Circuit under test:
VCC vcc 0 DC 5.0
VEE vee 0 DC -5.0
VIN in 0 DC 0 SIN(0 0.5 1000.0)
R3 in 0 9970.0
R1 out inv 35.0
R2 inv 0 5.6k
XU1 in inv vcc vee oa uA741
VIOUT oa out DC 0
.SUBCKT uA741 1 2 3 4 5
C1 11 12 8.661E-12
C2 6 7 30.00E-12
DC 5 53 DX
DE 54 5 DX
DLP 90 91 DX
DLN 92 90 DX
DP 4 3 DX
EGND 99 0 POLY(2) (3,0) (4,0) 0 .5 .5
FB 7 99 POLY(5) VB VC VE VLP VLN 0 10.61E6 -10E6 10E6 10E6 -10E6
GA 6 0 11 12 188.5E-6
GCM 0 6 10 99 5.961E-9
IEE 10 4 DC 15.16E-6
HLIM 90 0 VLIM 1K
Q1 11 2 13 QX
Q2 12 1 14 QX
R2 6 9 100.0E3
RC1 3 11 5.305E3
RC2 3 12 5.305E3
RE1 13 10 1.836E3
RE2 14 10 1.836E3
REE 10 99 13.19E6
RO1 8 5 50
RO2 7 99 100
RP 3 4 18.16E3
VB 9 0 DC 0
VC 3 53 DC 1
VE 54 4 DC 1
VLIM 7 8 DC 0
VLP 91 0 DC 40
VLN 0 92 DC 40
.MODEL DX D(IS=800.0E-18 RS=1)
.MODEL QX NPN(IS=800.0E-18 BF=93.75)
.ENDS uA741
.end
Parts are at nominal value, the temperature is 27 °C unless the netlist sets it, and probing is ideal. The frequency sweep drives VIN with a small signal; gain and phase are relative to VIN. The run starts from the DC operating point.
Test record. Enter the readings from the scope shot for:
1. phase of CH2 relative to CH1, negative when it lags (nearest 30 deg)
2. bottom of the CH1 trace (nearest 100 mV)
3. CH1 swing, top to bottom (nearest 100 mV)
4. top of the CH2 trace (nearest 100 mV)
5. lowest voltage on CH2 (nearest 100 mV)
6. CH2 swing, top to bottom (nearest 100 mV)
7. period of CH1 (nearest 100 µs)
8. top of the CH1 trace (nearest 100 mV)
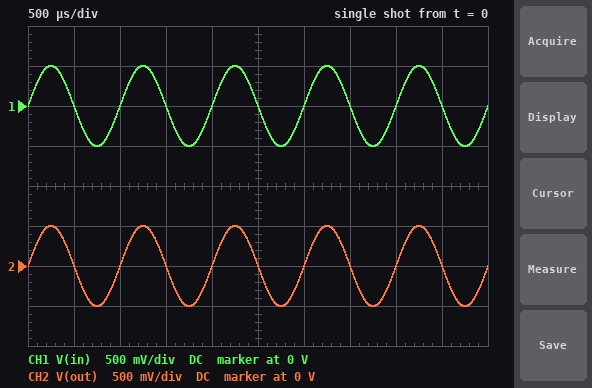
0 deg
-500 mV
1.0 V
500 mV
-500 mV
1.0 V
1.0 ms
500 mV
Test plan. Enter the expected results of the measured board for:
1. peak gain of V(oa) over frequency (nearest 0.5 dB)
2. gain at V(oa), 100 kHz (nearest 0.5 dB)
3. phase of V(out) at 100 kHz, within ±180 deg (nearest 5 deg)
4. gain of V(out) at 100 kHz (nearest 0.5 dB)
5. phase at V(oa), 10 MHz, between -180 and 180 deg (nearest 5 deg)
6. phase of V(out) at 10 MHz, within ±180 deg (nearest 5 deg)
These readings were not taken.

0 dB
0 dB
-5 deg
0 dB
-170 deg
-170 deg
